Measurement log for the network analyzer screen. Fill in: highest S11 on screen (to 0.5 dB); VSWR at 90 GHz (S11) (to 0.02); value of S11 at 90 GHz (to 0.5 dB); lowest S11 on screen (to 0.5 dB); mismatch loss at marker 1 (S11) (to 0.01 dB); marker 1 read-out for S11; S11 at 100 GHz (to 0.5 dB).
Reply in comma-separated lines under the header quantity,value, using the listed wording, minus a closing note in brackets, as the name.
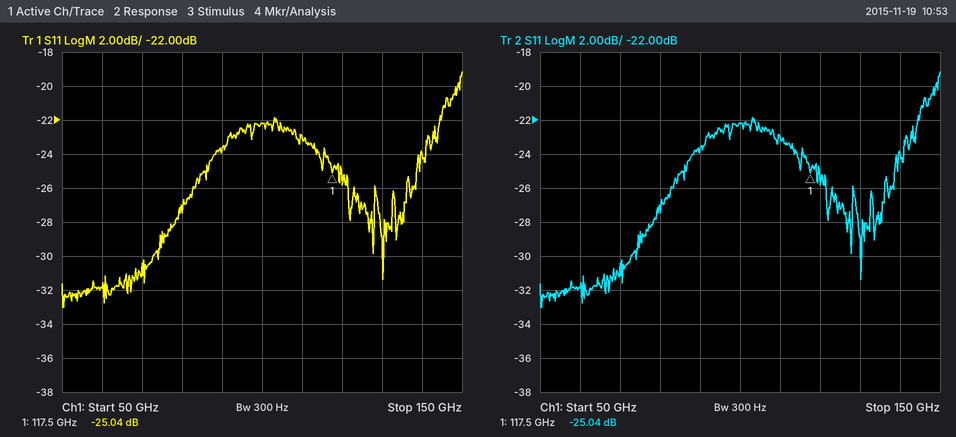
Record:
quantity,value
highest S11 on screen,-19.0 dB
VSWR at 90 GHz (S11),1.14
value of S11 at 90 GHz,-23.5 dB
lowest S11 on screen,-33.0 dB
mismatch loss at marker 1 (S11),0.01 dB
marker 1 read-out for S11,-25.04 dB
S11 at 100 GHz,-22.0 dB
